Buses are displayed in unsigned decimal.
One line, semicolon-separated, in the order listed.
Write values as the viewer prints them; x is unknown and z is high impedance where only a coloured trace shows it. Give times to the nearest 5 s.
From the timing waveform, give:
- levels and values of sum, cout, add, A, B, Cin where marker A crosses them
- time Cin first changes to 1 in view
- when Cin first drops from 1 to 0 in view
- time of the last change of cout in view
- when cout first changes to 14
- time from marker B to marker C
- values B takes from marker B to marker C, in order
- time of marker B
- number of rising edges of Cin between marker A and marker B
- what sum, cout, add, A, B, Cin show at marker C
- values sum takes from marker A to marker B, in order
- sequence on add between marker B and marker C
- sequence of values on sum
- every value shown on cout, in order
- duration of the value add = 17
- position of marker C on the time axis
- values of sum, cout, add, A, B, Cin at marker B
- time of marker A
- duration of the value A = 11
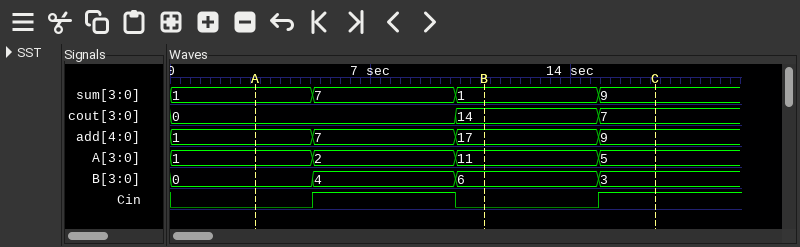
sum=1, cout=0, add=1, A=1, B=0, Cin=0; 5 s; 10 s; 15 s; 10 s; 5 s; 6, 3; 10 s; 1; sum=9, cout=7, add=9, A=5, B=3, Cin=1; 1, 7, 1; 17, 9; 1, 7, 1, 9; 0, 14, 7; 5 s; 15 s; sum=1, cout=14, add=17, A=11, B=6, Cin=0; 5 s; 5 s
